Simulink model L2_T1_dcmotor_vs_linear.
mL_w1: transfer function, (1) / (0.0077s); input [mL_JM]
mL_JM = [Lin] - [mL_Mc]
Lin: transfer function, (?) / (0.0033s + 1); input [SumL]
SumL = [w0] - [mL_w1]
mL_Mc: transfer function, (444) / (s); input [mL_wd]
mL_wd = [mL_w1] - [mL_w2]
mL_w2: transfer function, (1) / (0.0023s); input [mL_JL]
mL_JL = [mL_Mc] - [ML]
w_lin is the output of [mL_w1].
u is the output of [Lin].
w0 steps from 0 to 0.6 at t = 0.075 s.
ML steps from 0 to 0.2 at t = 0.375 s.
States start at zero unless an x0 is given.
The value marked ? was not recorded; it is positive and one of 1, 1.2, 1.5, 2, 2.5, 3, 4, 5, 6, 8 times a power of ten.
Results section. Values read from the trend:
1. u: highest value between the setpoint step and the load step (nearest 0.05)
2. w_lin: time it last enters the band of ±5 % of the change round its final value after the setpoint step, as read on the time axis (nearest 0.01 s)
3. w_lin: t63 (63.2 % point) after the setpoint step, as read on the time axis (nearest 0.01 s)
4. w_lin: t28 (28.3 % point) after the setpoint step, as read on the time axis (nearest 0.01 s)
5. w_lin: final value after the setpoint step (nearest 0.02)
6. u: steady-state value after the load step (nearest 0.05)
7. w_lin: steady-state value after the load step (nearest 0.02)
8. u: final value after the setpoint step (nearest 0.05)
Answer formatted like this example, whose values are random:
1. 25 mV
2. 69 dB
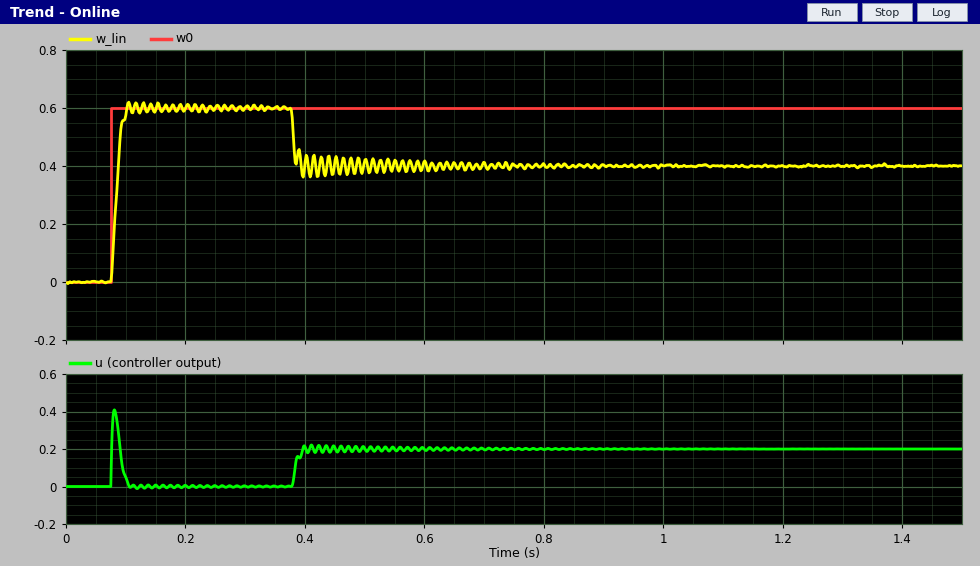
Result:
1. 0.40
2. 0.10 s
3. 0.09 s
4. 0.08 s
5. 0.60
6. 0.20
7. 0.40
8. 0.00
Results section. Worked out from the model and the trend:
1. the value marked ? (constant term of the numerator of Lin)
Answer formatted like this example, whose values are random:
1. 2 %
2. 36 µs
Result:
1. 1
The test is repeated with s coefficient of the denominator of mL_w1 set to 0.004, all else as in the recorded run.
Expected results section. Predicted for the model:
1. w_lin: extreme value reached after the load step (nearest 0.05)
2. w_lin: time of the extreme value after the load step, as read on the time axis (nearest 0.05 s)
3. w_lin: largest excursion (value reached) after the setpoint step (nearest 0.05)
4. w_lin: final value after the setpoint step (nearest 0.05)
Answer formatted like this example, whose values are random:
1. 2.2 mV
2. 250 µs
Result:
1. 0.35
2. 0.40 s
3. 0.65
4. 0.60
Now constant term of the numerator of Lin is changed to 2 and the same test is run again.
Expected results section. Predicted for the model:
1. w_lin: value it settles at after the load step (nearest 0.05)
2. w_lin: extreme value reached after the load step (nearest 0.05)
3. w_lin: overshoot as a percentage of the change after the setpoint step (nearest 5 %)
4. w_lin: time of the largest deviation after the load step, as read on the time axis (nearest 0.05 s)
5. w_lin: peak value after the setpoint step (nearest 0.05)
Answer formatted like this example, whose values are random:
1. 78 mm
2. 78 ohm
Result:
1. 0.50
2. 0.45
3. 15 %
4. 0.40 s
5. 0.70
